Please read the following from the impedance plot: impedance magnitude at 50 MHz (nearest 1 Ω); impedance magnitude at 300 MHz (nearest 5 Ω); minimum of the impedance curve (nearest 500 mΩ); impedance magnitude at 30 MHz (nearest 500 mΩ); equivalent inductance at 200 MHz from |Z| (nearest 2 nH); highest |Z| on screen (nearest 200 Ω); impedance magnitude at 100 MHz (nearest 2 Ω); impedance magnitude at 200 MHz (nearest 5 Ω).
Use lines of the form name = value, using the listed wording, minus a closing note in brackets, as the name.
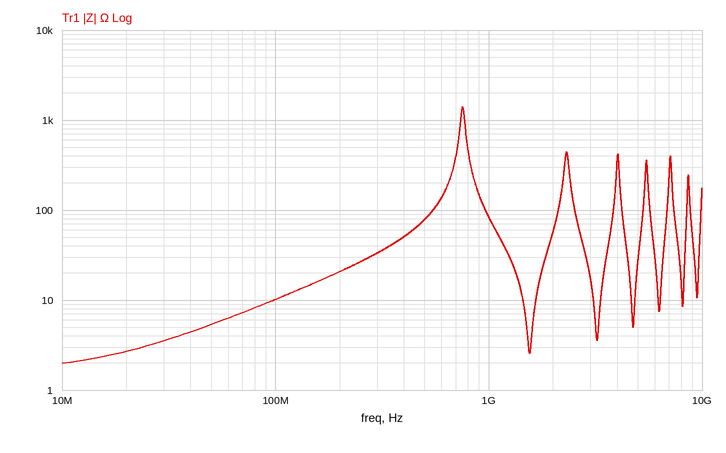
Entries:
impedance magnitude at 50 MHz = 5 Ω
impedance magnitude at 300 MHz = 35 Ω
minimum of the impedance curve = 2.0 Ω
impedance magnitude at 30 MHz = 3.5 Ω
equivalent inductance at 200 MHz from |Z| = 16 nH
highest |Z| on screen = 1.4 kΩ
impedance magnitude at 100 MHz = 10 Ω
impedance magnitude at 200 MHz = 20 Ω
